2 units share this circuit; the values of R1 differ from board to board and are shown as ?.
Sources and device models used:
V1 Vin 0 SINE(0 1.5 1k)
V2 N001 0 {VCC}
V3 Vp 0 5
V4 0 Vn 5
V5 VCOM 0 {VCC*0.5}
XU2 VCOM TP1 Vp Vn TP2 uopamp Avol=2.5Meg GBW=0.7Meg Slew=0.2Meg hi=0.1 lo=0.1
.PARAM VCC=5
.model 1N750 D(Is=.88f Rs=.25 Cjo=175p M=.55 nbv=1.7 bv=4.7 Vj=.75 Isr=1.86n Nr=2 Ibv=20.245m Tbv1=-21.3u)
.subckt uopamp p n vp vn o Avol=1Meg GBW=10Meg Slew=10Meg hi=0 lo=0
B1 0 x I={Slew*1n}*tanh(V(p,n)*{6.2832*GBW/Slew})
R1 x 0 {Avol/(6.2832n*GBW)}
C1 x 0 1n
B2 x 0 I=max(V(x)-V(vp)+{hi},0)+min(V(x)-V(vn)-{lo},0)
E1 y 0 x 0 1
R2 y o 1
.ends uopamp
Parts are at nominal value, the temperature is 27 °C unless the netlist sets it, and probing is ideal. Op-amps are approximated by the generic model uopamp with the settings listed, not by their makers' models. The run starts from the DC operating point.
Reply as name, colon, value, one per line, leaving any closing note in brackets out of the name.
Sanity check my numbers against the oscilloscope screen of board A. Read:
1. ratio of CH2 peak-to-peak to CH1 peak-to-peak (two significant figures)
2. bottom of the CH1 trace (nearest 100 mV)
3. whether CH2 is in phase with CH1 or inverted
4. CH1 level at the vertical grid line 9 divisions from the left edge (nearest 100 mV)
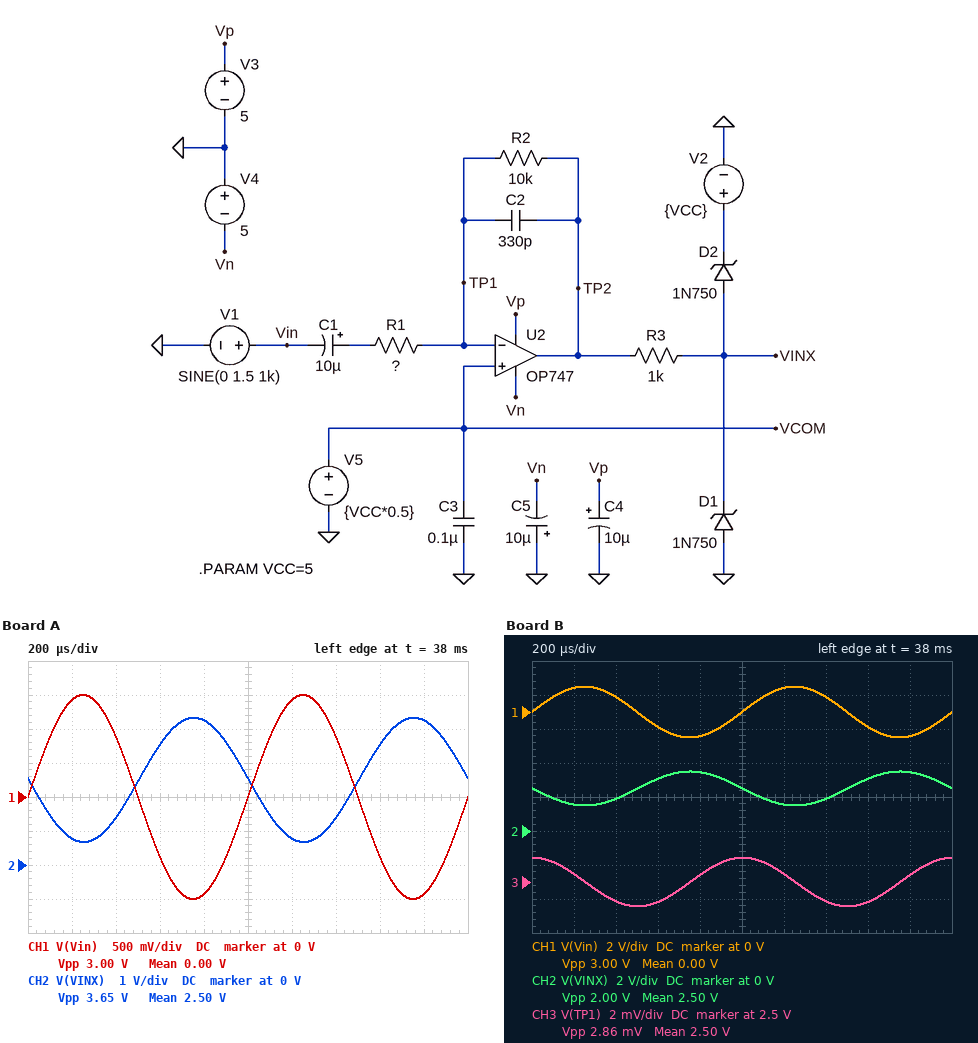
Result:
ratio of CH2 peak-to-peak to CH1 peak-to-peak: 1.2
bottom of the CH1 trace: -1.5 V
whether CH2 is in phase with CH1 or inverted: inverted
CH1 level at the vertical grid line 9 divisions from the left edge: -1.4 V
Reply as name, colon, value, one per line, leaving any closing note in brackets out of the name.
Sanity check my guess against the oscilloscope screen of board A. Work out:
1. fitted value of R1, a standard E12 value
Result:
fitted value of R1, a standard E12 value: 8.2 kΩ
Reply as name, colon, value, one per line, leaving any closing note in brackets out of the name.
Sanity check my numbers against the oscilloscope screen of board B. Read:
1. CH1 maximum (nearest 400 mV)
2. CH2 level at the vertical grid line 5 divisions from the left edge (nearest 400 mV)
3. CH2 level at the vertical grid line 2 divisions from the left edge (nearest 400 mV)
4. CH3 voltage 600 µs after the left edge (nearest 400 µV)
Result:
CH1 maximum: 1.6 V
CH2 level at the vertical grid line 5 divisions from the left edge: 2.4 V
CH2 level at the vertical grid line 2 divisions from the left edge: 2.0 V
CH3 voltage 600 µs after the left edge: 2.4988 V
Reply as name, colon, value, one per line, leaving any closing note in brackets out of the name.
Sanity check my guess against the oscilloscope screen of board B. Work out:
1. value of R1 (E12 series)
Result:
value of R1: 15 kΩ
